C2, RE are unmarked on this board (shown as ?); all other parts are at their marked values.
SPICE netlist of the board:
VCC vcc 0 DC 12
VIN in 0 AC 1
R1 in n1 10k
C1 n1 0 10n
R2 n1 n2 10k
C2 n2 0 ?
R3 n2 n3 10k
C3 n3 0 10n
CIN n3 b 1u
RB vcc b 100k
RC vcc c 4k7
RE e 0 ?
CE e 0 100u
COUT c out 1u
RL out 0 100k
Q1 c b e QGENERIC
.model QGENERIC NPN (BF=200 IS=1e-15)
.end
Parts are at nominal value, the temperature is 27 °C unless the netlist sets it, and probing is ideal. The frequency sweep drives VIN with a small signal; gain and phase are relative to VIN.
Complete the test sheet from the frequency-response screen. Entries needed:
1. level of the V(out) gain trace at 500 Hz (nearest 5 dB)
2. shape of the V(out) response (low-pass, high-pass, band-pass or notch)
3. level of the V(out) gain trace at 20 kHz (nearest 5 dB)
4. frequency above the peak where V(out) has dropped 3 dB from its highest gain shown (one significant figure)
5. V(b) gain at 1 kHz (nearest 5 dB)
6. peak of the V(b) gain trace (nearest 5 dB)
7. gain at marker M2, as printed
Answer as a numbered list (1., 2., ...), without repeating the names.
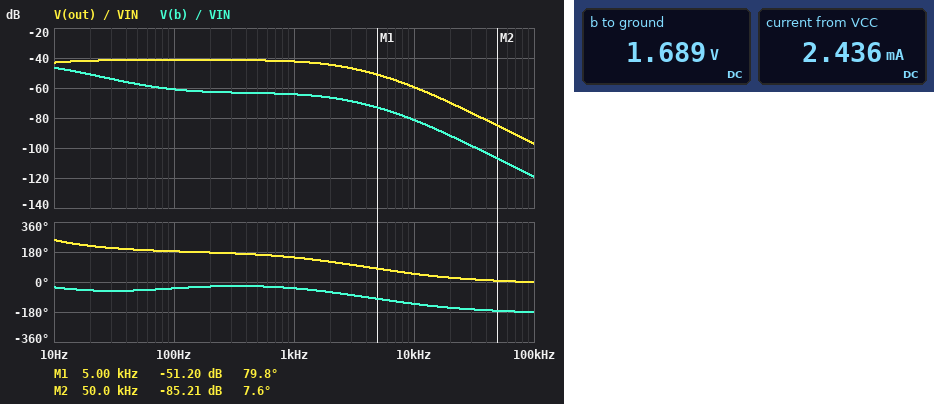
1. -40 dB
2. low-pass
3. -70 dB
4. 2 kHz
5. -65 dB
6. -45 dB
7. -85.21 dB
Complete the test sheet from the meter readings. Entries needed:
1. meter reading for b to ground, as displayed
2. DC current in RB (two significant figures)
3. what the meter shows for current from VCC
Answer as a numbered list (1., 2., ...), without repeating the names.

1. 1.689 V
2. 100 µA
3. 2.436 mA
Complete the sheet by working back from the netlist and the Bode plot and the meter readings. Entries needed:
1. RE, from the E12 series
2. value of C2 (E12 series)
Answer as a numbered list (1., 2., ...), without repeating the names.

1. 390 Ω
2. 4.7 nF
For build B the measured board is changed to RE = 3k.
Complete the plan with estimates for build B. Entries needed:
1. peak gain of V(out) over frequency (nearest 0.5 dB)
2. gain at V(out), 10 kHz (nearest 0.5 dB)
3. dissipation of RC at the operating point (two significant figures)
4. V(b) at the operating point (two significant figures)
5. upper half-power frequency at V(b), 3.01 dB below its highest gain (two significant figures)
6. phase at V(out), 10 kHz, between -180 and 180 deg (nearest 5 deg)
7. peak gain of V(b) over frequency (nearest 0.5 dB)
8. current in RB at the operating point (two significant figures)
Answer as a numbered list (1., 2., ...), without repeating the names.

1. -37.5 dB
2. -55.5 dB
3. 11 mW
4. 5.5 V
5. 7.0 Hz
6. 50 deg
7. -40.5 dB
8. 65 µA
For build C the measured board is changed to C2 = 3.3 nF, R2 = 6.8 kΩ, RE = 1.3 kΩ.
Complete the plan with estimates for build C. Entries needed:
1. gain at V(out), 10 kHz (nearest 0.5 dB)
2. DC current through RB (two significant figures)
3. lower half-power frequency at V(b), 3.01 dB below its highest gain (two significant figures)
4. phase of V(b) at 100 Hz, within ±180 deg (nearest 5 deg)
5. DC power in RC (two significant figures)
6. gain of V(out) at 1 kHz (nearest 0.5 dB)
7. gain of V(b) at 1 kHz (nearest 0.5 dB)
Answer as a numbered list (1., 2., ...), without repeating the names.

1. -54.0 dB
2. 86 µA
3. 1.1 Hz
4. -35 deg
5. 18 mW
6. -39.5 dB
7. -61.5 dB
